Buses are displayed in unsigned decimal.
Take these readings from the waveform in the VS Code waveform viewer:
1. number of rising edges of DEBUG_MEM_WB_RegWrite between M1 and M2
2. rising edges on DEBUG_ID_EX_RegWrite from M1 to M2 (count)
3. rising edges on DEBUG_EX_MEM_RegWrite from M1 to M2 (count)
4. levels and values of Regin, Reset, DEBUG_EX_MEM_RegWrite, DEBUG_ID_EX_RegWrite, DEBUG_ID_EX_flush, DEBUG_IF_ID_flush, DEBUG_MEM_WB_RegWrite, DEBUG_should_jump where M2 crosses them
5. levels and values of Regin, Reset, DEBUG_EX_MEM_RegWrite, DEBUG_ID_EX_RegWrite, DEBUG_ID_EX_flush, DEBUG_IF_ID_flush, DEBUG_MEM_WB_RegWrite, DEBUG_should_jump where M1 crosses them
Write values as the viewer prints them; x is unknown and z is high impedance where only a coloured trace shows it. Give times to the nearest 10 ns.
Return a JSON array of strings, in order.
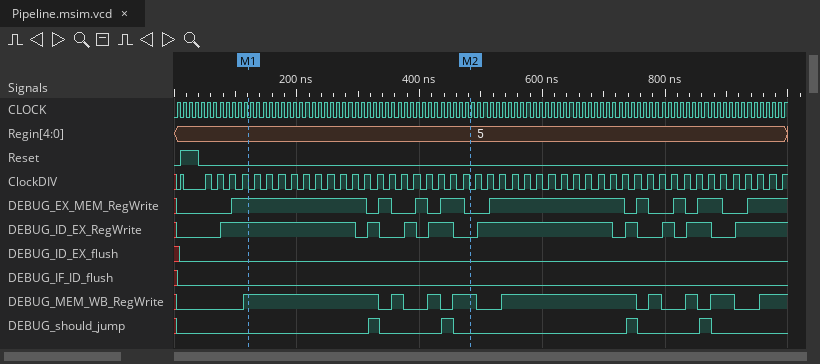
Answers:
["3", "3", "3", "Regin=5, Reset=0, DEBUG_EX_MEM_RegWrite=0, DEBUG_ID_EX_RegWrite=0, DEBUG_ID_EX_flush=0, DEBUG_IF_ID_flush=0, DEBUG_MEM_WB_RegWrite=1, DEBUG_should_jump=0", "Regin=5, Reset=0, DEBUG_EX_MEM_RegWrite=1, DEBUG_ID_EX_RegWrite=1, DEBUG_ID_EX_flush=0, DEBUG_IF_ID_flush=0, DEBUG_MEM_WB_RegWrite=1, DEBUG_should_jump=0"]
